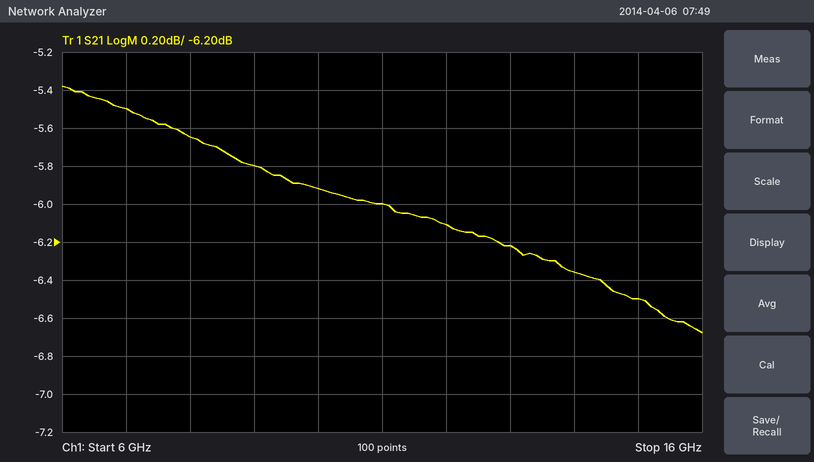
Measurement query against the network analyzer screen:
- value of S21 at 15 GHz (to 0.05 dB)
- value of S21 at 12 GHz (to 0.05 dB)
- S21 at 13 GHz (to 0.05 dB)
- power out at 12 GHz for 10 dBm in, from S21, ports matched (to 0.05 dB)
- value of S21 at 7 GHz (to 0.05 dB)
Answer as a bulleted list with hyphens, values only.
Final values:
- -6.50 dB
- -6.10 dB
- -6.20 dB
- 3.90 dBm
- -5.50 dB
